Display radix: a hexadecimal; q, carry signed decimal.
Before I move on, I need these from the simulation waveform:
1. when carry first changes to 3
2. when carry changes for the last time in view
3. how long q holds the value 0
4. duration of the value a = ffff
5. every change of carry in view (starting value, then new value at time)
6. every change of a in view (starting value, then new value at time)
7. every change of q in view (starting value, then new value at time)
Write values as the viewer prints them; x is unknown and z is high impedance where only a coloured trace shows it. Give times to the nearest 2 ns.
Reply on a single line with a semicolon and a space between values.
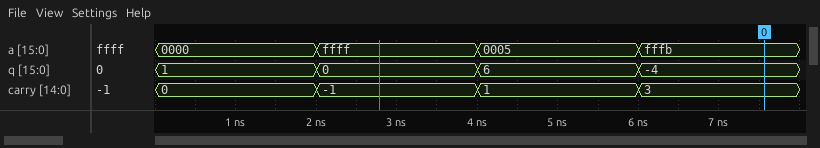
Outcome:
6 ns; 6 ns; 2 ns; 2 ns; 0, -1 at 2 ns, 1 at 4 ns, 3 at 6 ns; 0000, ffff at 2 ns, 0005 at 4 ns, fffb at 6 ns; 1, 0 at 2 ns, 6 at 4 ns, -4 at 6 ns
